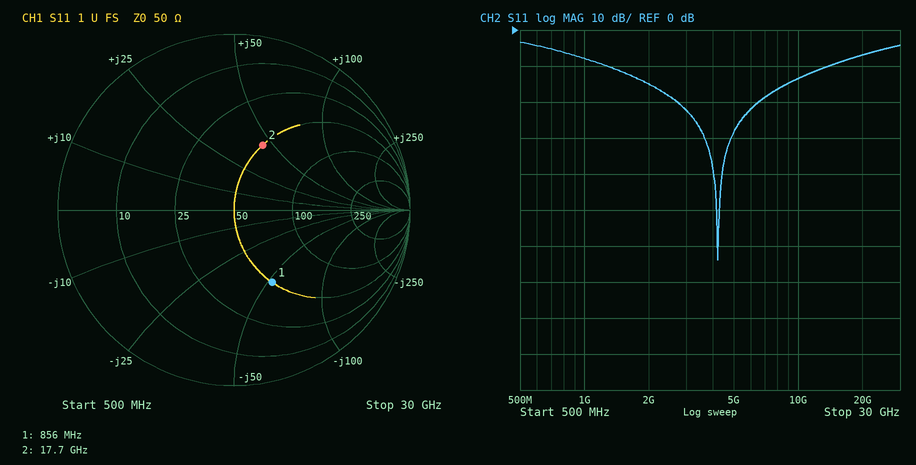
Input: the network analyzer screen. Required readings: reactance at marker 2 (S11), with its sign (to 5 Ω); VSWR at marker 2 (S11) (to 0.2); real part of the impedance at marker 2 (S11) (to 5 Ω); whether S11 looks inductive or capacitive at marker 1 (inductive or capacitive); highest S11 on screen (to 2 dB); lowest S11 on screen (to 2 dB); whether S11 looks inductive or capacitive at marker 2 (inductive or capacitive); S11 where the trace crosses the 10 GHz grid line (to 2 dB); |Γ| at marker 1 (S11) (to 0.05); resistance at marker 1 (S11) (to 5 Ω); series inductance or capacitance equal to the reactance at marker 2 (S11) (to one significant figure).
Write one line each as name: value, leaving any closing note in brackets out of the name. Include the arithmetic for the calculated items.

reactance at marker 2 (S11), with its sign: +45 Ω
VSWR at marker 2 (S11): 2.4
real part of the impedance at marker 2 (S11): 50 Ω
whether S11 looks inductive or capacitive at marker 1: capacitive
highest S11 on screen: -4 dB
lowest S11 on screen: -64 dB
whether S11 looks inductive or capacitive at marker 2: inductive
S11 where the trace crosses the 10 GHz grid line: -14 dB
|Γ| at marker 1 (S11): 0.45
resistance at marker 1 (S11): 50 Ω
series inductance or capacitance equal to the reactance at marker 2 (S11): L = 45 Ω/(2π × 17.7 GHz) ≈ 405 pH, so 400 pH to one significant figure
